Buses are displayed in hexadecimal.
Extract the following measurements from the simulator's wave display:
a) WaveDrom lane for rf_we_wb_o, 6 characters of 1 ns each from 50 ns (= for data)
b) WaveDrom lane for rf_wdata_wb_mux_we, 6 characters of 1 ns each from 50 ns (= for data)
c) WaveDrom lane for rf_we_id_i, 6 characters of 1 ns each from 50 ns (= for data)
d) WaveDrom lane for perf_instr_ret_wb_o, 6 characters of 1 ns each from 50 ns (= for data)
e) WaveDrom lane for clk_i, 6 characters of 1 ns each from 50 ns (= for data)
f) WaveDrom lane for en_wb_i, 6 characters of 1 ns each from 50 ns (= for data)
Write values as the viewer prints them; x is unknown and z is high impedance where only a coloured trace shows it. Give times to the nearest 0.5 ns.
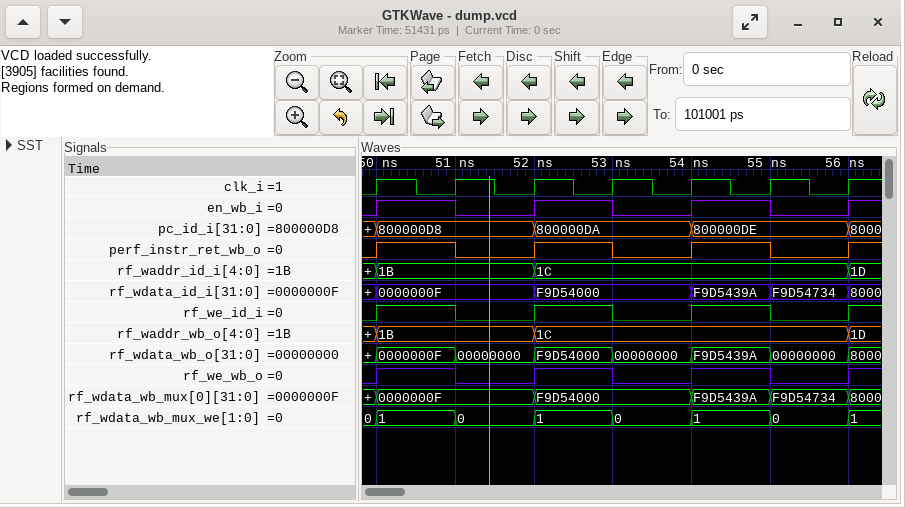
{name: 'rf_we_wb_o', wave: '101010'}
{name: 'rf_wdata_wb_mux_we', wave: '======', data: '1 0 1 0 1 0'}
{name: 'rf_we_id_i', wave: '101010'}
{name: 'perf_instr_ret_wb_o', wave: '101010'}
{name: 'clk_i', wave: 'p.....'}
{name: 'en_wb_i', wave: '101010'}
